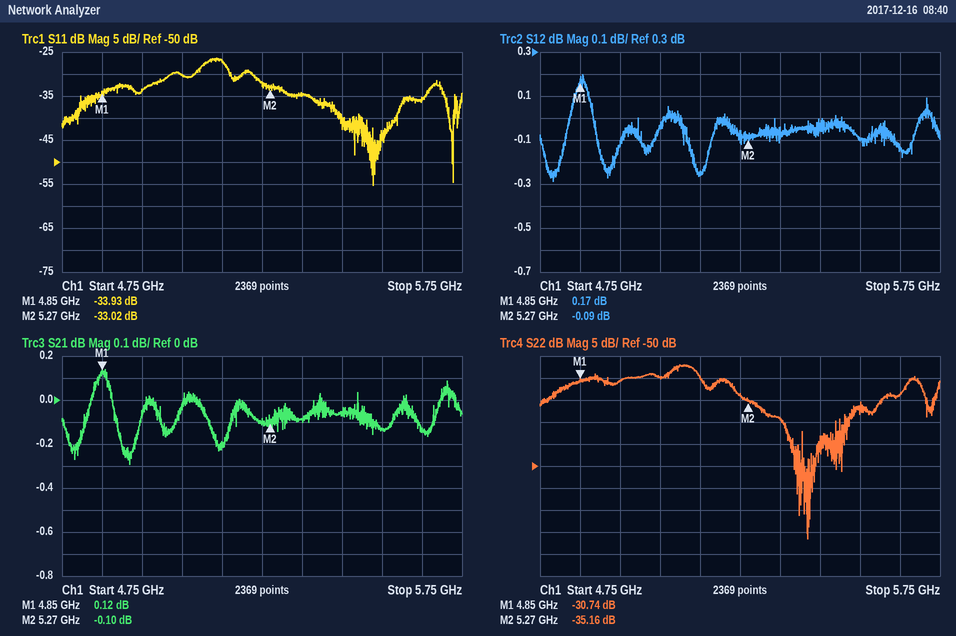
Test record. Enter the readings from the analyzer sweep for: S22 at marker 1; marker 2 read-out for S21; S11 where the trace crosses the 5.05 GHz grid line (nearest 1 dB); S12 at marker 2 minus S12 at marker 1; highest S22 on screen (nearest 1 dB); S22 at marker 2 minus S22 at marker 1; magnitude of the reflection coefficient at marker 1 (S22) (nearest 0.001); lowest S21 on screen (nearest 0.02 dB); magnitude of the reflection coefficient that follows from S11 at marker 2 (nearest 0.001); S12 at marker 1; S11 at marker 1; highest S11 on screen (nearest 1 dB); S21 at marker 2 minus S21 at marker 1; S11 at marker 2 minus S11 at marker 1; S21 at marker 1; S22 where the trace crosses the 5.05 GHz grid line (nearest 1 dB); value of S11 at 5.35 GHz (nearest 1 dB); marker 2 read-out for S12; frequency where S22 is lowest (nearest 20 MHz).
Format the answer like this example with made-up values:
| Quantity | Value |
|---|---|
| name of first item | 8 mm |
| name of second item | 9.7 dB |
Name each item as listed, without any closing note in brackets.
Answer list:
| Quantity | Value |
|---|---|
| S22 at marker 1 | -30.74 dB |
| marker 2 read-out for S21 | -0.10 dB |
| S11 where the trace crosses the 5.05 GHz grid line | -30 dB |
| S12 at marker 2 minus S12 at marker 1 | -0.26 dB |
| highest S22 on screen | -27 dB |
| S22 at marker 2 minus S22 at marker 1 | -4.42 dB |
| magnitude of the reflection coefficient at marker 1 (S22) | 0.029 |
| lowest S21 on screen | -0.30 dB |
| magnitude of the reflection coefficient that follows from S11 at marker 2 | 0.022 |
| S12 at marker 1 | 0.17 dB |
| S11 at marker 1 | -33.93 dB |
| highest S11 on screen | -26 dB |
| S21 at marker 2 minus S21 at marker 1 | -0.22 dB |
| S11 at marker 2 minus S11 at marker 1 | 0.91 dB |
| S21 at marker 1 | 0.12 dB |
| S22 where the trace crosses the 5.05 GHz grid line | -30 dB |
| value of S11 at 5.35 GHz | -35 dB |
| marker 2 read-out for S12 | -0.09 dB |
| frequency where S22 is lowest | 5.42 GHz |
